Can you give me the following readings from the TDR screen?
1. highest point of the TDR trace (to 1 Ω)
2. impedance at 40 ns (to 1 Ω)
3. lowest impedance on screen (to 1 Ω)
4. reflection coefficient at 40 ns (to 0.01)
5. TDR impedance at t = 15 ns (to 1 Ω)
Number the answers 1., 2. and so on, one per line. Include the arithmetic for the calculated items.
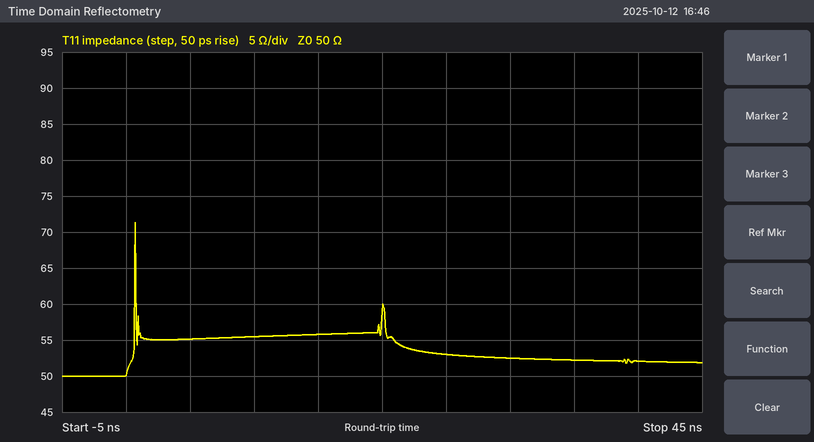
1. 71 Ω
2. 52 Ω
3. 50 Ω
4. (52 − 50)/(52 + 50) ≈ +0.02
5. 56 Ω
